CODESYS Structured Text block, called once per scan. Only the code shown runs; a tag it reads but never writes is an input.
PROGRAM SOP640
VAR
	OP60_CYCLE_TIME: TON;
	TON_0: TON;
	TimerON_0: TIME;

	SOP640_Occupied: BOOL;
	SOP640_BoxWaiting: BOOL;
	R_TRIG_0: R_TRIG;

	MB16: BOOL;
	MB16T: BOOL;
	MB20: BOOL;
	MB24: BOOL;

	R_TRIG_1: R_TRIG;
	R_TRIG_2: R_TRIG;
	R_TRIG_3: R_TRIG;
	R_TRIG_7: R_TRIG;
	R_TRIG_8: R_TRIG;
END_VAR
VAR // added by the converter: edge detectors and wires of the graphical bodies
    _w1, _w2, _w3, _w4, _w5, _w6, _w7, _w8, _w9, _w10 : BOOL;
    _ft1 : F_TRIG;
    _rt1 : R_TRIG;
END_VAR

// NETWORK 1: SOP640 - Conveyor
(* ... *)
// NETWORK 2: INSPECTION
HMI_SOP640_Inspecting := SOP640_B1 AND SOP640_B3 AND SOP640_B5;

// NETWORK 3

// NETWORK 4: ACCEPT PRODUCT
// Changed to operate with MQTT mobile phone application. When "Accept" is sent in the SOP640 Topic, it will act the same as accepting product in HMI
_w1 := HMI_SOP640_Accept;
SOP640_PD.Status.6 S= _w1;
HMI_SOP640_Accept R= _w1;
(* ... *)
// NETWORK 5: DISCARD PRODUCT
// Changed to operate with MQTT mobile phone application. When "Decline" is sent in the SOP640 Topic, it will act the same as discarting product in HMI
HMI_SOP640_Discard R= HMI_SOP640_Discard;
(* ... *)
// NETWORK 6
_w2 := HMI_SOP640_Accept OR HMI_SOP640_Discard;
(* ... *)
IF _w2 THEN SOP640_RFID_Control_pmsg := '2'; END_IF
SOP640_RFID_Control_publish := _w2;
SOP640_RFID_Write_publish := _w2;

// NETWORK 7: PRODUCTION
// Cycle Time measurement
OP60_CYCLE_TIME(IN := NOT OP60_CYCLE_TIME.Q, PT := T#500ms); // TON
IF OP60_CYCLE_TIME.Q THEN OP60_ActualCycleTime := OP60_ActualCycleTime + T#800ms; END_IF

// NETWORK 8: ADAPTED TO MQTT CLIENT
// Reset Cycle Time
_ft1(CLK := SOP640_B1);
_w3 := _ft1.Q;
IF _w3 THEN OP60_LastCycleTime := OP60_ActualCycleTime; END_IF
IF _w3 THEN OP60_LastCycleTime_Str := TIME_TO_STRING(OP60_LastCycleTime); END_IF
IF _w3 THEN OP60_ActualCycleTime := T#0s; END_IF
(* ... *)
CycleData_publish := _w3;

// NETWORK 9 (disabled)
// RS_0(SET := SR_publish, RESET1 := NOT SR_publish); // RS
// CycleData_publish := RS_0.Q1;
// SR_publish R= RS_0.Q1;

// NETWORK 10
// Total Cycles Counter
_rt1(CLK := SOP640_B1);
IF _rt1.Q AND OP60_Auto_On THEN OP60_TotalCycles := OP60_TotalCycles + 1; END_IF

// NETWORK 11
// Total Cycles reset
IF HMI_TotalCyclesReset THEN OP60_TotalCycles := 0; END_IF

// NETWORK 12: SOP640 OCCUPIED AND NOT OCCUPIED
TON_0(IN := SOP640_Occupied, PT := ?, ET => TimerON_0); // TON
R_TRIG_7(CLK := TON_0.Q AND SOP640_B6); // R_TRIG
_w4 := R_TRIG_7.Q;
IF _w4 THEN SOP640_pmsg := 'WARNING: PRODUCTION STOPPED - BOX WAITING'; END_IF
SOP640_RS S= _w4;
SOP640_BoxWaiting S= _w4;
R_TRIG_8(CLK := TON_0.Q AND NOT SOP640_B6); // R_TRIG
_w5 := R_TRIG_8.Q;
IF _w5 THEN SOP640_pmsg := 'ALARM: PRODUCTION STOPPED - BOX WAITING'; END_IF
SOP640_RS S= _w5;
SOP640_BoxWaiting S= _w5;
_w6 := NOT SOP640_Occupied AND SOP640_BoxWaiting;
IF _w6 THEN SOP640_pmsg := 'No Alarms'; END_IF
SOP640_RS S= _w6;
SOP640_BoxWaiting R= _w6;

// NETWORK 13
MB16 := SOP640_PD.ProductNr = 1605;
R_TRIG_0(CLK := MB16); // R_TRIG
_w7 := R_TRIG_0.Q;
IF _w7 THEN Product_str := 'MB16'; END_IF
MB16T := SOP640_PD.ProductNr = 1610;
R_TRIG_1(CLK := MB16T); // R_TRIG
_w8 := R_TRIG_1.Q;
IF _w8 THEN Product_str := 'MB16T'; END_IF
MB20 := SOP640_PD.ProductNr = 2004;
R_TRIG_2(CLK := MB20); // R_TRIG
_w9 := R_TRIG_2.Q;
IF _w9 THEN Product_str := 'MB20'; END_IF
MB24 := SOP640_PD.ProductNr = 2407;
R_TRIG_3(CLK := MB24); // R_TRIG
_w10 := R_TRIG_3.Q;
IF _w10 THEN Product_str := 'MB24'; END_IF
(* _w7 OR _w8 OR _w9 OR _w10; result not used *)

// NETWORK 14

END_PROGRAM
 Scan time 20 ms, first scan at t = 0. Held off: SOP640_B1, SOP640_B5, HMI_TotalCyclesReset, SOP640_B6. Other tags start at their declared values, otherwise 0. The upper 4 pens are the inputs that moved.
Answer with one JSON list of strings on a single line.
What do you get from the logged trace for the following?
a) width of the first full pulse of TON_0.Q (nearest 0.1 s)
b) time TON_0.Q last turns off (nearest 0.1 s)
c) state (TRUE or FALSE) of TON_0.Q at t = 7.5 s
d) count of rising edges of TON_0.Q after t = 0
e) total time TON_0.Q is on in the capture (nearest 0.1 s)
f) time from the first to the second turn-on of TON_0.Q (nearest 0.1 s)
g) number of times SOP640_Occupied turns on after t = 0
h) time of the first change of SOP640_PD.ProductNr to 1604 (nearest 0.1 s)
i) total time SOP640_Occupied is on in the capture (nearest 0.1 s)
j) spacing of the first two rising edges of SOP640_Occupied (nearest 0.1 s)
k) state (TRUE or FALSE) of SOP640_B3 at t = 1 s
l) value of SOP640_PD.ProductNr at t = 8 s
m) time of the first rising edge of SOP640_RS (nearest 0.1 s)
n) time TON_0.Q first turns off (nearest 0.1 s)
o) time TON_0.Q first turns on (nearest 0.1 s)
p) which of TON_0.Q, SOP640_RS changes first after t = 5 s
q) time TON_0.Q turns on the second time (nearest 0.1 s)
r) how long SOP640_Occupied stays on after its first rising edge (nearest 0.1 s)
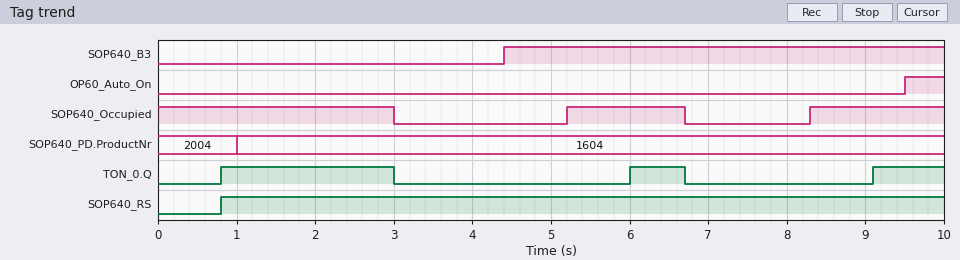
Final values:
["2.2 s", "6.7 s", "FALSE", "3", "3.8 s", "5.2 s", "2", "1.0 s", "6.2 s", "3.1 s", "FALSE", "1604", "0.8 s", "3.0 s", "0.8 s", "TON_0.Q", "6.0 s", "1.5 s"]
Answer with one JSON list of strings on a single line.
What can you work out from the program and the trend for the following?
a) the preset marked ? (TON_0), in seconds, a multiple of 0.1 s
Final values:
["0.8 s"]
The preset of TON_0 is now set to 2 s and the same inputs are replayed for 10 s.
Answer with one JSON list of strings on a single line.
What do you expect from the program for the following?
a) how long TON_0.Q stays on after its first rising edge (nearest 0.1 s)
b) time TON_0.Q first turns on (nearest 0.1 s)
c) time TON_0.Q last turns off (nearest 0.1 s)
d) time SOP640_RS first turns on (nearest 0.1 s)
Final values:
["1.0 s", "2.0 s", "3.0 s", "2.0 s"]
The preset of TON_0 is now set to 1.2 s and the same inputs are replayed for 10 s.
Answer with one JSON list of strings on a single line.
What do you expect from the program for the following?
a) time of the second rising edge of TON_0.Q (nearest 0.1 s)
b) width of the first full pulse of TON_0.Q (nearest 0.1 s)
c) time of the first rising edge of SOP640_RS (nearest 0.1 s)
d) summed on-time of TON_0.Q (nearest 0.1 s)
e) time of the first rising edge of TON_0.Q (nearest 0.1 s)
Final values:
["6.4 s", "1.8 s", "1.2 s", "2.6 s", "1.2 s"]
